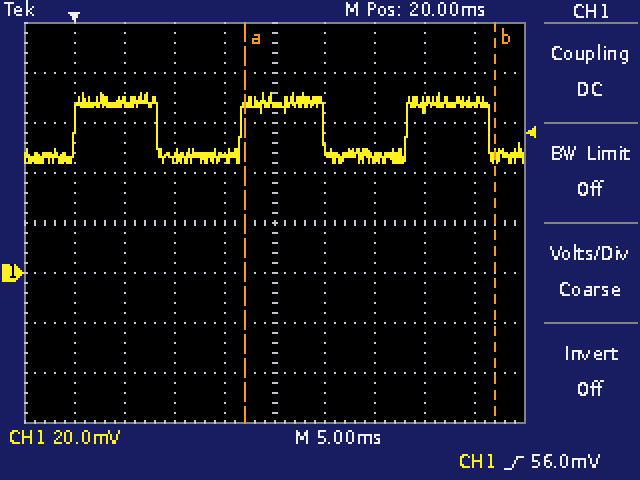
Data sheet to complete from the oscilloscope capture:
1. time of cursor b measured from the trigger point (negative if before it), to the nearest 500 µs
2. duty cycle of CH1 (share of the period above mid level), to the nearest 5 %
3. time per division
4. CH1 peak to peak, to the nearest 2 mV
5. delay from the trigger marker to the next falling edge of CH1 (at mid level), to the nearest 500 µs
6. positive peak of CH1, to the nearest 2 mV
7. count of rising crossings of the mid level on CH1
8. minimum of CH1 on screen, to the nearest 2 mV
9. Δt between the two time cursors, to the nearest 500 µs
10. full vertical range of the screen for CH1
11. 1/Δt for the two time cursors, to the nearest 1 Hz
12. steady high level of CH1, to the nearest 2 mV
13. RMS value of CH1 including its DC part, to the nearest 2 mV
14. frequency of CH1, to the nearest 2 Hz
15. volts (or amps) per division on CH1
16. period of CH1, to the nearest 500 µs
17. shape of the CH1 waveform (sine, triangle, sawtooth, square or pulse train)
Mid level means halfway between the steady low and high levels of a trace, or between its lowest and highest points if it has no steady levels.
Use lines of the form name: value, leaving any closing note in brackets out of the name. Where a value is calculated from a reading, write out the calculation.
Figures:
time of cursor b measured from the trigger point (negative if before it), to the nearest 500 µs: +42.0 ms
duty cycle of CH1 (share of the period above mid level), to the nearest 5 %: 50 %
time per division: 5 ms
CH1 peak to peak, to the nearest 2 mV: 72 mV − (44 mV) = 28 mV
delay from the trigger marker to the next falling edge of CH1 (at mid level), to the nearest 500 µs: 8.5 ms
positive peak of CH1, to the nearest 2 mV: 72 mV
count of rising crossings of the mid level on CH1: 3
minimum of CH1 on screen, to the nearest 2 mV: 44 mV
Δt between the two time cursors, to the nearest 500 µs: 25.0 ms
full vertical range of the screen for CH1: 160 mV
1/Δt for the two time cursors, to the nearest 1 Hz: 1 / 25.0 ms ≈ 40 Hz
steady high level of CH1, to the nearest 2 mV: 68 mV
RMS value of CH1 including its DC part, to the nearest 2 mV: √(0.5 × (68 mV)² + 0.5 × (44 mV)²) ≈ 57.3 mV, so 58 mV to the nearest 2 mV
frequency of CH1, to the nearest 2 Hz: 1 / 16.5 ms ≈ 60.6 Hz, so 60 Hz to the nearest 2 Hz
volts (or amps) per division on CH1: 20 mV
period of CH1, to the nearest 500 µs: 16.5 ms
shape of the CH1 waveform: square
